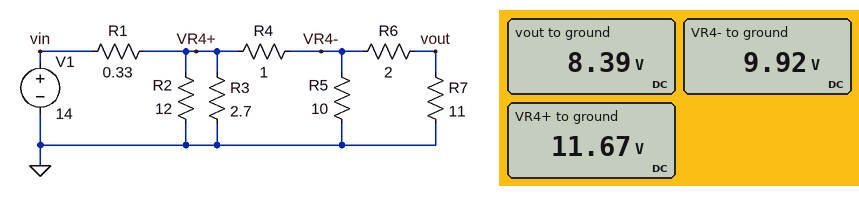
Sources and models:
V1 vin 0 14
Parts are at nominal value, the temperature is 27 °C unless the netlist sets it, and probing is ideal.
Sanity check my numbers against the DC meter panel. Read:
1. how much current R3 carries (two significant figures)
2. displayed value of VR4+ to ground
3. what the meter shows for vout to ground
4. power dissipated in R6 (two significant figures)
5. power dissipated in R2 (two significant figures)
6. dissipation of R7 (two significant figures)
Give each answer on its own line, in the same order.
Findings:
4.3 A
11.67 V
8.39 V
1.2 W
11 W
6.4 W
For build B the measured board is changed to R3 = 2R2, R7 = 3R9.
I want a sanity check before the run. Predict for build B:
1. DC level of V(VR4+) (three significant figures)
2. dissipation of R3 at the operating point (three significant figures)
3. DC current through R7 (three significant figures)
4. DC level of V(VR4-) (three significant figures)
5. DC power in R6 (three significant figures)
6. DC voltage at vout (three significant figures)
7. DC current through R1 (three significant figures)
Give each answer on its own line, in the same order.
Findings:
11.2 V
57.2 W
1.50 A
8.84 V
4.49 W
5.84 V
8.42 A
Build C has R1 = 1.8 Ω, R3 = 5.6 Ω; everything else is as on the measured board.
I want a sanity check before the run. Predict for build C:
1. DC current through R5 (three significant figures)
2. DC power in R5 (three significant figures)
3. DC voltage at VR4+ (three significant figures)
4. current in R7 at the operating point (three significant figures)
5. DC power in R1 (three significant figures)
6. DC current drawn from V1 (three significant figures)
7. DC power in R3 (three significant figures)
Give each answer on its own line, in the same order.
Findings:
683 mA
4.66 W
8.04 V
525 mA
19.8 W
3.31 A
11.5 W
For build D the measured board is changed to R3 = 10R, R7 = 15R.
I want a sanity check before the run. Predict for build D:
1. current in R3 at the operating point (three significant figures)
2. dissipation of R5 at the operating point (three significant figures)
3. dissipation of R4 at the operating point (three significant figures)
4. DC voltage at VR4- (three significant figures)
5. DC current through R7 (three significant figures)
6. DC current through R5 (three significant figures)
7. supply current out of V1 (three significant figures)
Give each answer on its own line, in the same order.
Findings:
1.27 A
11.9 W
3.01 W
10.9 V
643 mA
1.09 A
4.06 A
